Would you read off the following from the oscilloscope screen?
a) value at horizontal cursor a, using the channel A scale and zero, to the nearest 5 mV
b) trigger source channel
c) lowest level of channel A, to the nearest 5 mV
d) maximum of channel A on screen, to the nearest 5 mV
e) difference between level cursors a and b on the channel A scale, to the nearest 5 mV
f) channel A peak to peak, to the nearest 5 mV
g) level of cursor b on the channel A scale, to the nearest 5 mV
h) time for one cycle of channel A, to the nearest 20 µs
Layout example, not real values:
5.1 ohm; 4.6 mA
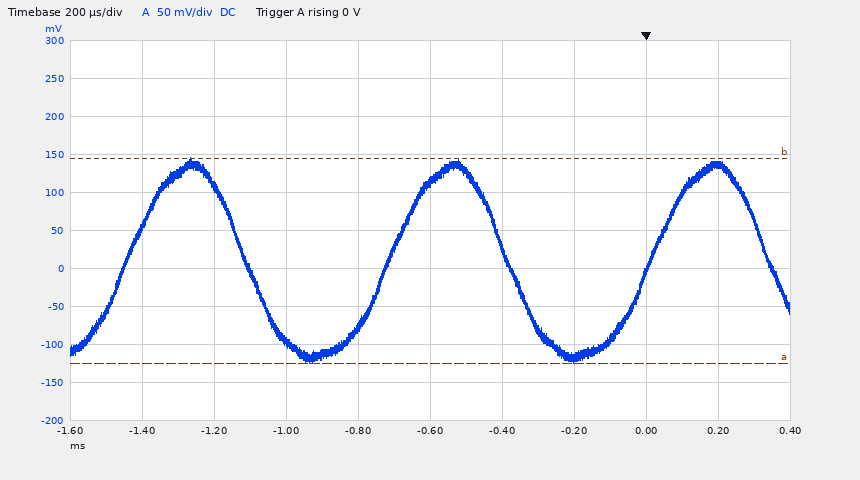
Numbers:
-125 mV; channel A; -125 mV; 145 mV; 270 mV; 270 mV; 145 mV; 720 µs
